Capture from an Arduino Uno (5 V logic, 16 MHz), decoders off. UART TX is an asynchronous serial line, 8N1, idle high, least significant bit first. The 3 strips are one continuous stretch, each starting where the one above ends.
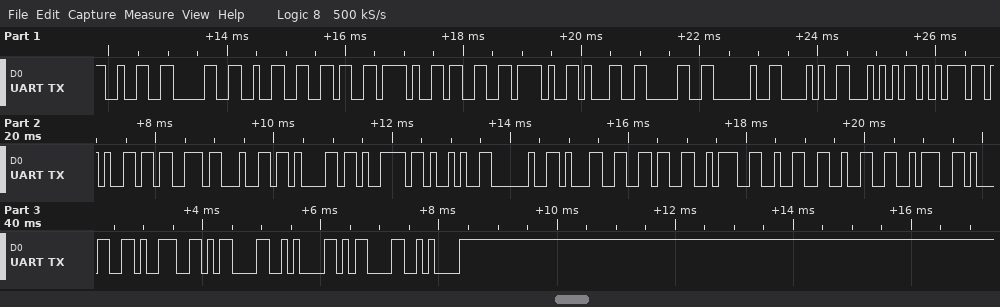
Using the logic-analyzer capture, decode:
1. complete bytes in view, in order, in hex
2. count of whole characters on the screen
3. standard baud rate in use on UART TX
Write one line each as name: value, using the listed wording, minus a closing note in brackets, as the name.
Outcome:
complete bytes in view, in order, in hex: 32 30 32 36 2F 33 2F 31 30 20 28 54 75 65 73 64 61 79 29 20 31 36 3A 32 32 3A 31 39 0D 0A 0D 0A
count of whole characters on the screen: 32
standard baud rate in use on UART TX: 9600 baud
